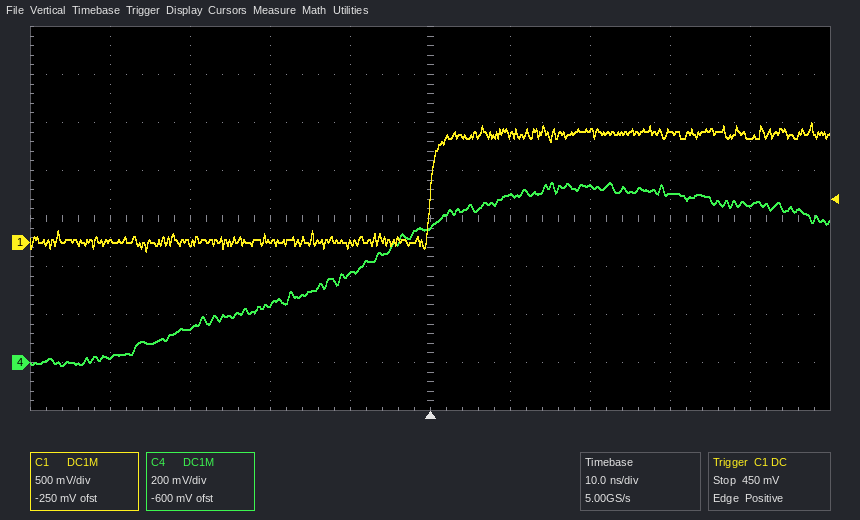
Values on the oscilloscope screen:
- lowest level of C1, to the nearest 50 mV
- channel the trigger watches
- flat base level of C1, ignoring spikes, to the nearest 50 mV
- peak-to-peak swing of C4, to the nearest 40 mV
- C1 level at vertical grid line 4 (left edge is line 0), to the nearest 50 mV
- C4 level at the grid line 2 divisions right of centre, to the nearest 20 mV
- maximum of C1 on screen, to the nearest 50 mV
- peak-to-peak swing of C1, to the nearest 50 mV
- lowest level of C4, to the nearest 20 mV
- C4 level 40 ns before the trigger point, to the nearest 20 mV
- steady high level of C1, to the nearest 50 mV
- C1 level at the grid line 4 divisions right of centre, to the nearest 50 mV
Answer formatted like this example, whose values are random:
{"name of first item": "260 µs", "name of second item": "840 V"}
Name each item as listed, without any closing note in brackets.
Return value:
{"lowest level of C1, to the nearest 50 mV": "-100 mV", "channel the trigger watches": "C1", "flat base level of C1, ignoring spikes, to the nearest 50 mV": "0 mV", "peak-to-peak swing of C4, to the nearest 40 mV": "760 mV", "C1 level at vertical grid line 4 (left edge is line 0), to the nearest 50 mV": "0 mV", "C4 level at the grid line 2 divisions right of centre, to the nearest 20 mV": "740 mV", "maximum of C1 on screen, to the nearest 50 mV": "1.25 V", "peak-to-peak swing of C1, to the nearest 50 mV": "1.35 V", "lowest level of C4, to the nearest 20 mV": "-20 mV", "C4 level 40 ns before the trigger point, to the nearest 20 mV": "20 mV", "steady high level of C1, to the nearest 50 mV": "1.15 V", "C1 level at the grid line 4 divisions right of centre, to the nearest 50 mV": "1.10 V"}
